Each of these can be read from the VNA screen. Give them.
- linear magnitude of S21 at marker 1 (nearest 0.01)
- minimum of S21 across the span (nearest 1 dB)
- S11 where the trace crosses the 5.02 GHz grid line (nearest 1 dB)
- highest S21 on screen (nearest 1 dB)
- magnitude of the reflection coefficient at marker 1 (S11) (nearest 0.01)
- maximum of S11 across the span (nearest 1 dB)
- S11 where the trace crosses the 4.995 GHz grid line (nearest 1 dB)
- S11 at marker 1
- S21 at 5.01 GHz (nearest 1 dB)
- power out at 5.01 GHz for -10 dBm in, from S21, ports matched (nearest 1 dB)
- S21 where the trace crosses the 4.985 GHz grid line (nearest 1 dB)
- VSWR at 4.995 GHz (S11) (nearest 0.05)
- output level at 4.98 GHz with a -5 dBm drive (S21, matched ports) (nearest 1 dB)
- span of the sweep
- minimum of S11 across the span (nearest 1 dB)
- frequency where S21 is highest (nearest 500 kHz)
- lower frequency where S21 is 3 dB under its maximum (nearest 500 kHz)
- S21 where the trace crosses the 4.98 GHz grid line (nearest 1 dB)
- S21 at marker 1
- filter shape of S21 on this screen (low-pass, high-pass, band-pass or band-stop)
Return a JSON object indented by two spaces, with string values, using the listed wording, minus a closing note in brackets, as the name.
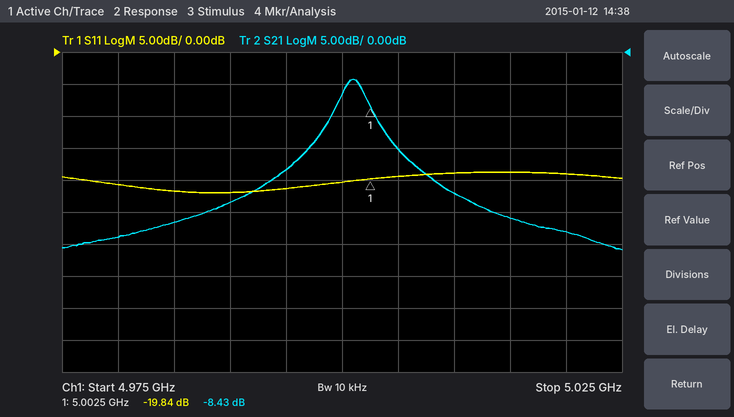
{
  "linear magnitude of S21 at marker 1": "0.38",
  "minimum of S21 across the span": "-31 dB",
  "S11 where the trace crosses the 5.02 GHz grid line": "-19 dB",
  "highest S21 on screen": "-4 dB",
  "magnitude of the reflection coefficient at marker 1 (S11)": "0.10",
  "maximum of S11 across the span": "-19 dB",
  "S11 where the trace crosses the 4.995 GHz grid line": "-21 dB",
  "S11 at marker 1": "-19.84 dB",
  "S21 at 5.01 GHz": "-22 dB",
  "power out at 5.01 GHz for -10 dBm in, from S21, ports matched": "-32 dBm",
  "S21 where the trace crosses the 4.985 GHz grid line": "-27 dB",
  "VSWR at 4.995 GHz (S11)": "1.20",
  "output level at 4.98 GHz with a -5 dBm drive (S21, matched ports)": "-34 dBm",
  "span of the sweep": "50 MHz",
  "minimum of S11 across the span": "-22 dB",
  "frequency where S21 is highest": "5.0010 GHz",
  "lower frequency where S21 is 3 dB under its maximum": "5.0000 GHz",
  "S21 where the trace crosses the 4.98 GHz grid line": "-29 dB",
  "S21 at marker 1": "-8.43 dB",
  "filter shape of S21 on this screen": "band-pass"
}
